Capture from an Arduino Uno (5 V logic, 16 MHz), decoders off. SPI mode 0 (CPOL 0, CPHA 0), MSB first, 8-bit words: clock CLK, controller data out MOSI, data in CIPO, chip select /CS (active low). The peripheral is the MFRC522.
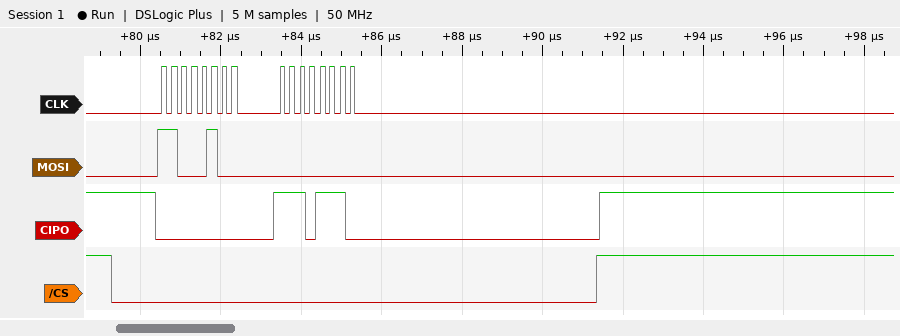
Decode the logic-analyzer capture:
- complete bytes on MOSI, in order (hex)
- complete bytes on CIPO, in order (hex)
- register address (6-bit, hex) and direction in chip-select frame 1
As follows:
C4 00
00 EE
0x22 read
